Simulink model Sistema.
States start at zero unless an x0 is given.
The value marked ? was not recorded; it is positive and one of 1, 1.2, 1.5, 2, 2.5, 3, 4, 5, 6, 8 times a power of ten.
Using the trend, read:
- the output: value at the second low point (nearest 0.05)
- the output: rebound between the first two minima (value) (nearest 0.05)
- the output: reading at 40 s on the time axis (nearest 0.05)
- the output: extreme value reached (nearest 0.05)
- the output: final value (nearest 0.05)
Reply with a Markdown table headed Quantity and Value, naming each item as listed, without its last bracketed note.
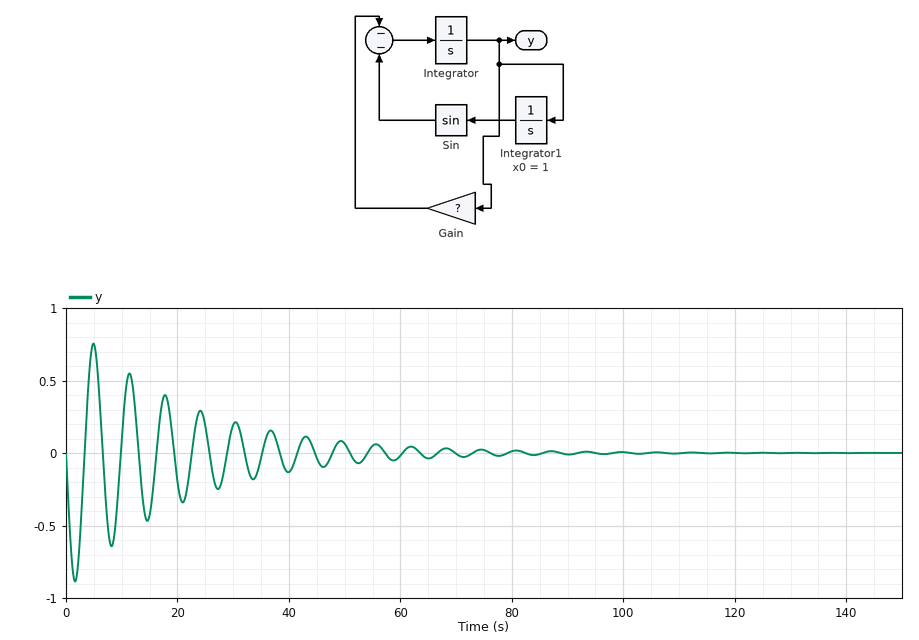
| Quantity | Value |
|---|---|
| the output: value at the second low point | -0.65 |
| the output: rebound between the first two minima (value) | 0.75 |
| the output: reading at 40 s on the time axis | -0.15 |
| the output: extreme value reached | -0.90 |
| the output: final value | 0.00 |
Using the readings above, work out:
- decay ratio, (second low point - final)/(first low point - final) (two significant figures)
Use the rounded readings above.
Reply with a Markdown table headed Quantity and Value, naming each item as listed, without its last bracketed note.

| Quantity | Value |
|---|---|
| decay ratio, (second low point - final)/(first low point - final) | 0.72 |
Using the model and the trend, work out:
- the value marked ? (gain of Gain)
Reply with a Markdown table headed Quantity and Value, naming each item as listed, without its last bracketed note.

| Quantity | Value |
|---|---|
| the value marked ? | 0.1 |
